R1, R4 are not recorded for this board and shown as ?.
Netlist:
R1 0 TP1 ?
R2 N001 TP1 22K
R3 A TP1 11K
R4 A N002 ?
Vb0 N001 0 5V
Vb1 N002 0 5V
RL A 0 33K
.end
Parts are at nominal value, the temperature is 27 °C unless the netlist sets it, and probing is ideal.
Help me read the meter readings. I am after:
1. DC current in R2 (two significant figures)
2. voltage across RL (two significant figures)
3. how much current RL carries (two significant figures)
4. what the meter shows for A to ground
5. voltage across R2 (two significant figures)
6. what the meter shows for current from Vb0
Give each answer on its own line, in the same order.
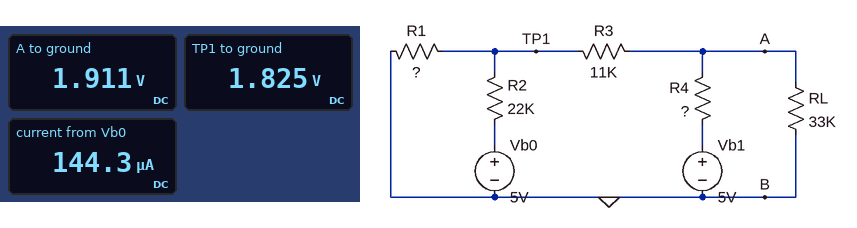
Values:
140 µA
1.9 V
58 µA
1.911 V
3.2 V
144.3 µA
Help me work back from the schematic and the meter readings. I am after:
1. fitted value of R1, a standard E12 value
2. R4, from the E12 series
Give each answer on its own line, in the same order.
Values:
12 kΩ
47 kΩ
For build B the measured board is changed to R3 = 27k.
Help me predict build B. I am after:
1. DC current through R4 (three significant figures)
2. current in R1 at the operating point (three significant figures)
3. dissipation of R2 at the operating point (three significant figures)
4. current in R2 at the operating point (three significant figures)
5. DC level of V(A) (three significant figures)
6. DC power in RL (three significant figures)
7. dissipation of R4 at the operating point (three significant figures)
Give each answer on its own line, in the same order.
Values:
64.8 µA
151 µA
463 µW
145 µA
1.96 V
116 µW
197 µW
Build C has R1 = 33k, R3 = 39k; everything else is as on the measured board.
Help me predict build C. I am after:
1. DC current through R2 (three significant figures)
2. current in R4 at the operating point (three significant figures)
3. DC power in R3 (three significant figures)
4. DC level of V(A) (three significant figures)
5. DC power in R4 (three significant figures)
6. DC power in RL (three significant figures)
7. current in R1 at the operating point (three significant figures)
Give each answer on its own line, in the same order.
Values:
98.8 µA
57.1 µA
6.69 µW
2.32 V
153 µW
163 µW
85.7 µA
